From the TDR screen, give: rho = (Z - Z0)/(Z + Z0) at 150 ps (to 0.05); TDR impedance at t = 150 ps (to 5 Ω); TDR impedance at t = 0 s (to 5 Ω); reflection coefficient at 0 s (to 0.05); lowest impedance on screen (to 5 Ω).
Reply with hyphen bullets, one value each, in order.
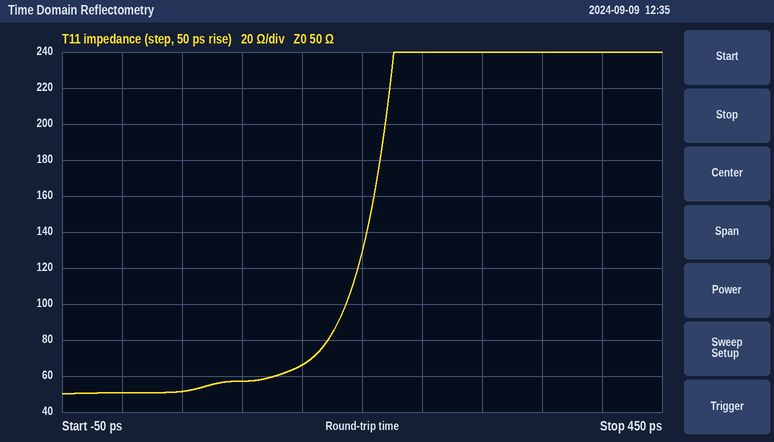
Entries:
- +0.15
- 65 Ω
- 50 Ω
- 0.00
- 50 Ω
